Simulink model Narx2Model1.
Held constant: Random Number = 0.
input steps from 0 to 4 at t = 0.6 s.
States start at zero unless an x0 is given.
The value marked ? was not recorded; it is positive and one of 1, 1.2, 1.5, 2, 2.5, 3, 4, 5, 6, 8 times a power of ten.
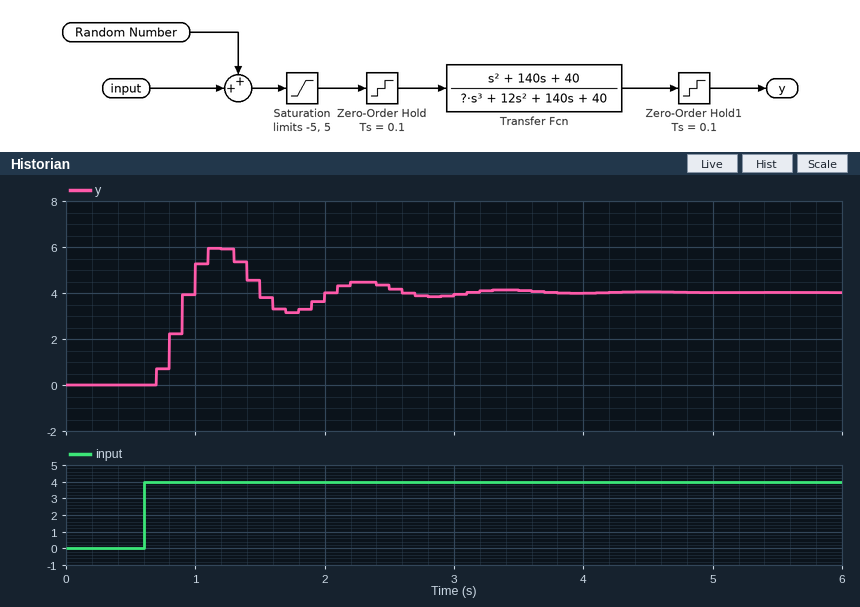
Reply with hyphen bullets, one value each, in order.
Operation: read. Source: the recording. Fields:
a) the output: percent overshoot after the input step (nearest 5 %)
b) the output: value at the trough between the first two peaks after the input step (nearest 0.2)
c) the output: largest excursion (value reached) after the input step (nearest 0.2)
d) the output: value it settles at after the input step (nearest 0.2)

- 50 %
- 3.2
- 6.0
- 4.0
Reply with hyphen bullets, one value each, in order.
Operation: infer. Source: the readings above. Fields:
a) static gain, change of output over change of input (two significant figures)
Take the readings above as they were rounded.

- 1.0
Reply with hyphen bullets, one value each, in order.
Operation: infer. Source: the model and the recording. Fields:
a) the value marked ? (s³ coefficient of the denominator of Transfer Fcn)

- 4
